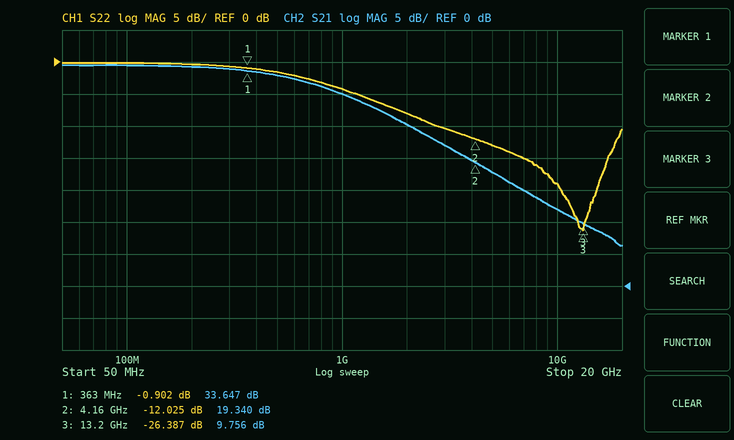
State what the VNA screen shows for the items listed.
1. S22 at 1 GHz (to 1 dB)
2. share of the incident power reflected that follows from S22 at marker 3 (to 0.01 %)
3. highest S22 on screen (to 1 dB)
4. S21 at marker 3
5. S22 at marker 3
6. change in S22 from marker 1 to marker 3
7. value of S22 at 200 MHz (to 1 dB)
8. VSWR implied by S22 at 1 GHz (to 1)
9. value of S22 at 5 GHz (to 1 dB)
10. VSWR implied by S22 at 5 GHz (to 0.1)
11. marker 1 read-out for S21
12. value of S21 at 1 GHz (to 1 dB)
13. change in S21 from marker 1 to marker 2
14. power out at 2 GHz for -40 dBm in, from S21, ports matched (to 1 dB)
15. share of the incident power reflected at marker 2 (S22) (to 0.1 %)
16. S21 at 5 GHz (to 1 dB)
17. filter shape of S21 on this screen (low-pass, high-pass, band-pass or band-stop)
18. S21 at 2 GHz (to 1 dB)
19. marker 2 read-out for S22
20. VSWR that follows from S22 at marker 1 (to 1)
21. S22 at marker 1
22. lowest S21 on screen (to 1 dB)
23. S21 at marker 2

-4 dB
0.23 %
0 dB
9.756 dB
-26.387 dB
-25.485 dB
0 dB
4
-13 dB
1.6
33.647 dB
30 dB
-14.307 dB
-15 dBm
6.3 %
18 dB
low-pass
25 dB
-12.025 dB
19
-0.902 dB
6 dB
19.340 dB
